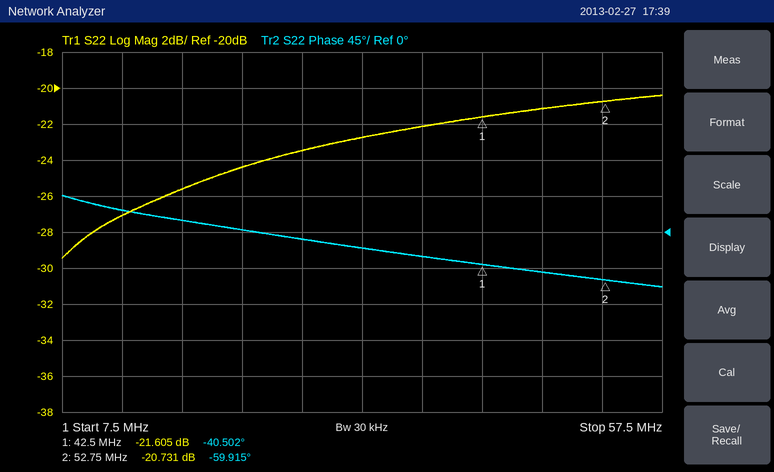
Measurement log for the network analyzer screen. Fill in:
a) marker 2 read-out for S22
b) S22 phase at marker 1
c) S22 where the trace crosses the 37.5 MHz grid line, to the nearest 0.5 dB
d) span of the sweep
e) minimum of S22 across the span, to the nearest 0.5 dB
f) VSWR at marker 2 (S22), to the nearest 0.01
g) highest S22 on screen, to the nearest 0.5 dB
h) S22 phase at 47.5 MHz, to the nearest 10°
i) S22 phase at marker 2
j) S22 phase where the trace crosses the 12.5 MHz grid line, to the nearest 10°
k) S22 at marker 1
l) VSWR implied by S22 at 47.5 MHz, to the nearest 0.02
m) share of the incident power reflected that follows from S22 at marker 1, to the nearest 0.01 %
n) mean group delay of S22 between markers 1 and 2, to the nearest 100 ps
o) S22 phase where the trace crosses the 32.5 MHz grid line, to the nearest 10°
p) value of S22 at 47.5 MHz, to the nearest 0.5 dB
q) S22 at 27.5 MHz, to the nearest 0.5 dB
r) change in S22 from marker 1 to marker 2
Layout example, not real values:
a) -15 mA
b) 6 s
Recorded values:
a) -20.731 dB
b) -40.502°
c) -22.0 dB
d) 50 MHz
e) -29.5 dB
f) 1.20
g) -20.5 dB
h) -50°
i) -59.915°
j) 30°
k) -21.605 dB
l) 1.20
m) 0.69 %
n) 5.3 ns
o) -20°
p) -21.0 dB
q) -23.5 dB
r) 0.874 dB
